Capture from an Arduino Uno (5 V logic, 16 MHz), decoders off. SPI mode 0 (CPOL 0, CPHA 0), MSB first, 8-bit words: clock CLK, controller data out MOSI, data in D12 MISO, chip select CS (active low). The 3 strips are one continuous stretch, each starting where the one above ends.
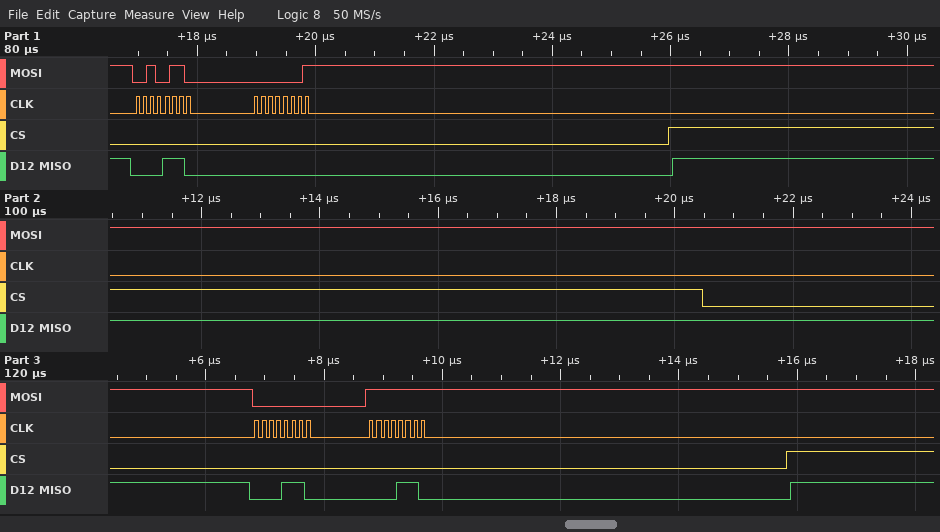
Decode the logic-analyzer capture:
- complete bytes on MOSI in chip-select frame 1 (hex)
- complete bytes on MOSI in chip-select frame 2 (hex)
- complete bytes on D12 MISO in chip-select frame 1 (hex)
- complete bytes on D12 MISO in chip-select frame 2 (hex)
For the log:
0x26 0x01
0x00 0xFF
0x0E 0x00
0x0E 0x0E
